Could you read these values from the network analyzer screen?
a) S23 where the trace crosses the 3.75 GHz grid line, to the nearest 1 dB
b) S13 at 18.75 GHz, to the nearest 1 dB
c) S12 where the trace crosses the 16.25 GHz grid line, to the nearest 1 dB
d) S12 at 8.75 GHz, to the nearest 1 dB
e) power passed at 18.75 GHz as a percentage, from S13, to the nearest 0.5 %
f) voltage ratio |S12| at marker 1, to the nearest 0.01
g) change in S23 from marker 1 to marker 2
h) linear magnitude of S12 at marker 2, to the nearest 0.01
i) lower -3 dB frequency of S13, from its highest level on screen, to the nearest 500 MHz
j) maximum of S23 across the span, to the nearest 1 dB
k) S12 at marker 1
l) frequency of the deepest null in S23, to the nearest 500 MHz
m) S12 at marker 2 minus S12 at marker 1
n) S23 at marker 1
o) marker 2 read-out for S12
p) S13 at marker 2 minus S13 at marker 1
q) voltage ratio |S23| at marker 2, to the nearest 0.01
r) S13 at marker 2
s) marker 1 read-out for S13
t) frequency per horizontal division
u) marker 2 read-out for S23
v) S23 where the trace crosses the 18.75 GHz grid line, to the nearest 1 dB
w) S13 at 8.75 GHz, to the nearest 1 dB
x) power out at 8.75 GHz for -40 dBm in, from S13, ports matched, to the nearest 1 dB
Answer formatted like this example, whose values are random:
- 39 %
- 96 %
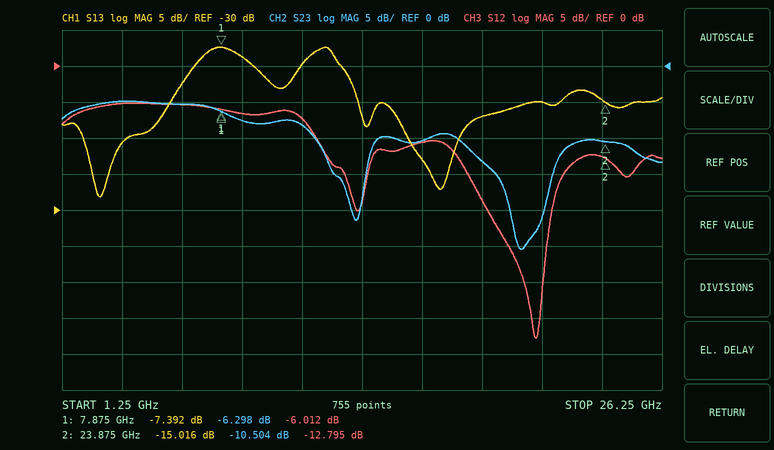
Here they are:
- -5 dB
- -17 dB
- -11 dB
- -7 dB
- 2.0 %
- 0.50
- -4.206 dB
- 0.23
- 6.5 GHz
- -5 dB
- -6.012 dB
- 20.5 GHz
- -6.783 dB
- -6.298 dB
- -12.795 dB
- -7.624 dB
- 0.30
- -15.016 dB
- -7.392 dB
- 2.5 GHz
- -10.504 dB
- -13 dB
- -9 dB
- -49 dBm
